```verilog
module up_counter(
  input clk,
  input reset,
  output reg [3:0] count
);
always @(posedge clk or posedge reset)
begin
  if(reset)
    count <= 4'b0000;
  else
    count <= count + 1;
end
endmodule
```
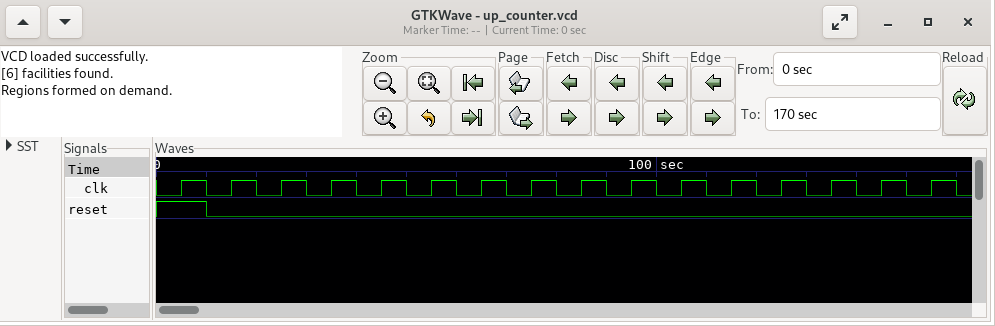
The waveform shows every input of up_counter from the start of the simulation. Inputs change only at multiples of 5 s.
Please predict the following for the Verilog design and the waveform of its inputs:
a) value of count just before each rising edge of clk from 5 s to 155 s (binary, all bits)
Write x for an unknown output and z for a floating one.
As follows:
0000, 0000, 0001, 0010, 0011, 0100, 0101, 0110, 0111, 1000, 1001, 1010, 1011, 1100, 1101, 1110
